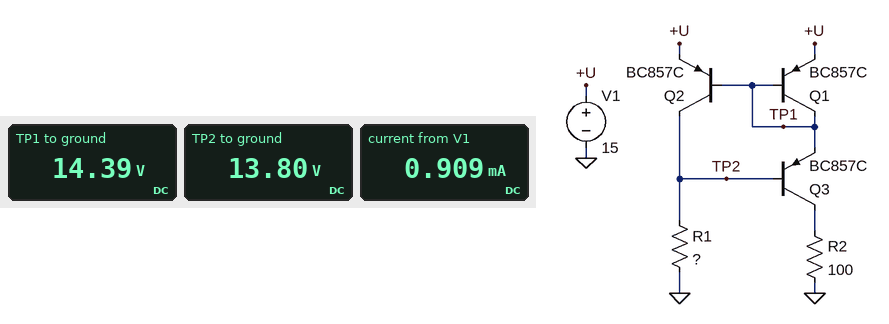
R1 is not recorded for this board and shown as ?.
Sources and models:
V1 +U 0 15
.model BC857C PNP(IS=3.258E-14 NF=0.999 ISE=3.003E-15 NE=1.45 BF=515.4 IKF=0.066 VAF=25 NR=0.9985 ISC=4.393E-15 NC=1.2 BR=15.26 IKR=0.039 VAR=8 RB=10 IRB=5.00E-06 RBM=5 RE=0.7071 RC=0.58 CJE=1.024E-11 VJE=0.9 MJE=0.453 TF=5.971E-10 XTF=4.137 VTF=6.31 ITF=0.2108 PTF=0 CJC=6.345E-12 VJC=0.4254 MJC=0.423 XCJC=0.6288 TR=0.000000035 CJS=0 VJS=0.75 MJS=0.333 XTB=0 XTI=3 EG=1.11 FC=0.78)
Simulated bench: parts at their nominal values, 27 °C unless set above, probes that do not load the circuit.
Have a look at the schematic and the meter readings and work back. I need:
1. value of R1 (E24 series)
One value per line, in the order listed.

30 kΩ
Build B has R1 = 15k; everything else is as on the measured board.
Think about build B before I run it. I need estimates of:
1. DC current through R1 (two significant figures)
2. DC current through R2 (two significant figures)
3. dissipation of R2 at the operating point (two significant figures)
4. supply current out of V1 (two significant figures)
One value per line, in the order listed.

920 µA
900 µA
80 µW
1.8 mA
